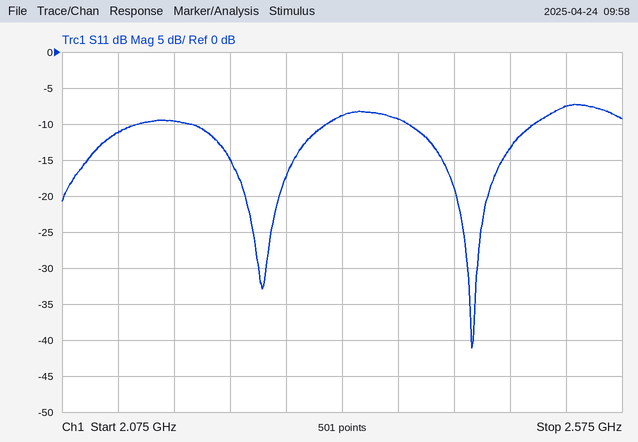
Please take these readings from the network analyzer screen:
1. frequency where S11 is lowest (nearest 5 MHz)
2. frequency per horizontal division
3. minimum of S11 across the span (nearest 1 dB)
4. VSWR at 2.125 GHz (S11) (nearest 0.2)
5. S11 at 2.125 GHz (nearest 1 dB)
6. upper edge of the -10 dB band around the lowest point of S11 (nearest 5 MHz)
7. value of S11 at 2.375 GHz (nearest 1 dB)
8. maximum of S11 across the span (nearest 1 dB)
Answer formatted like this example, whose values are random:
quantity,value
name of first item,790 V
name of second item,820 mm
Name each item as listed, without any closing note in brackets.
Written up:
quantity,value
frequency where S11 is lowest,2.440 GHz
frequency per horizontal division,50 MHz
minimum of S11 across the span,-41 dB
VSWR at 2.125 GHz (S11),1.8
S11 at 2.125 GHz,-11 dB
upper edge of the -10 dB band around the lowest point of S11,2.495 GHz
value of S11 at 2.375 GHz,-9 dB
maximum of S11 across the span,-7 dB
